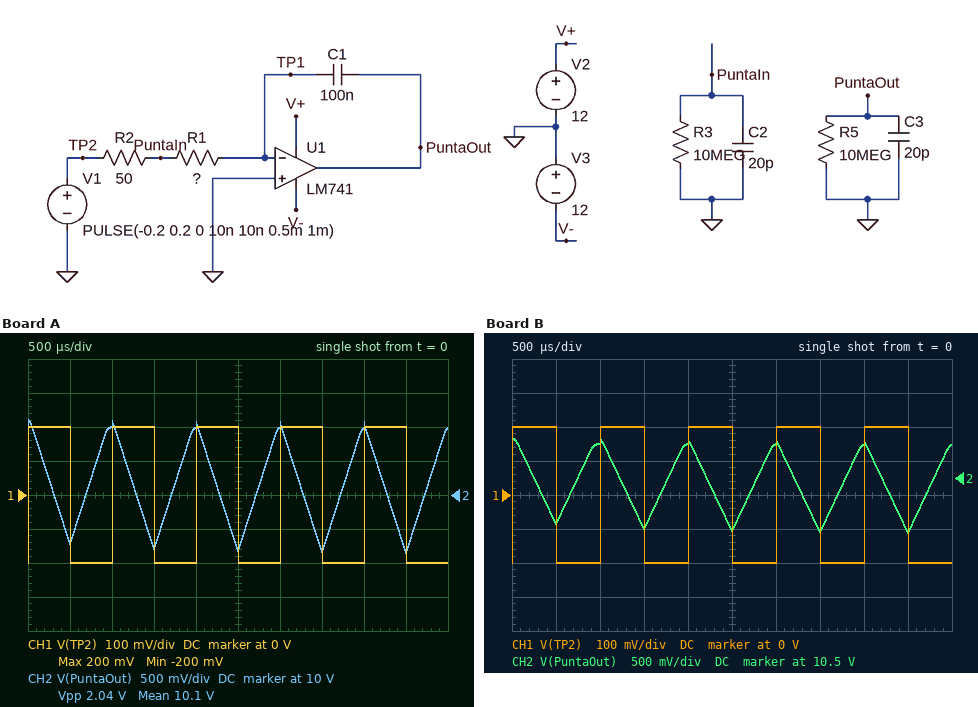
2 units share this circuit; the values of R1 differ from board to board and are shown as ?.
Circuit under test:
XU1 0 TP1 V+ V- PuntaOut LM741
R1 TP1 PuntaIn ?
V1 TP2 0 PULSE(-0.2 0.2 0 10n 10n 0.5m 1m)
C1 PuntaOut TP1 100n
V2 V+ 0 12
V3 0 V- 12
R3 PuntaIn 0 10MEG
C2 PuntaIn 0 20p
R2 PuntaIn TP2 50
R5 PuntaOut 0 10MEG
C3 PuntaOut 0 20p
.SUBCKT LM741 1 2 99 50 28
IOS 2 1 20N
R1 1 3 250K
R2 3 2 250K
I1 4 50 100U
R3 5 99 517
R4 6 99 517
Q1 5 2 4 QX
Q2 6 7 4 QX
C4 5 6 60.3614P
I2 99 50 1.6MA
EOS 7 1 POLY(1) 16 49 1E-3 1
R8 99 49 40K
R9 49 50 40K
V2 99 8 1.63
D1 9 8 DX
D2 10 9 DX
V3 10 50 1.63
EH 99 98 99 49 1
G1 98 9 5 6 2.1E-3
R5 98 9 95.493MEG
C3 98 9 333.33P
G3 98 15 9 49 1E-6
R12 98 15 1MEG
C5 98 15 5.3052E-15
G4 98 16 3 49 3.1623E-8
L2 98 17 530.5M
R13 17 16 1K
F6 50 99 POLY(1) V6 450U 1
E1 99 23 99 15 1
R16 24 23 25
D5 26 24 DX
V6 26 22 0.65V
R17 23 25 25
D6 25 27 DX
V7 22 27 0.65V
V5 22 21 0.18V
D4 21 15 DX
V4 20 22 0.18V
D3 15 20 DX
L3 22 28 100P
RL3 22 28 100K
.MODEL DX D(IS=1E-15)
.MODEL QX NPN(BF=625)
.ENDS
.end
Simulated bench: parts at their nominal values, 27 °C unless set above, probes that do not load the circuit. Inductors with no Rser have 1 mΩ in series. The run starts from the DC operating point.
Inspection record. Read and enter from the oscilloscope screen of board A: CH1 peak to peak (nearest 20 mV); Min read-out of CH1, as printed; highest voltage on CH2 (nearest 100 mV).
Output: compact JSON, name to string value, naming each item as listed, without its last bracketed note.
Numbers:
{"CH1 peak to peak": "400 mV", "Min read-out of CH1, as printed": "-200 mV", "highest voltage on CH2": "11.1 V"}
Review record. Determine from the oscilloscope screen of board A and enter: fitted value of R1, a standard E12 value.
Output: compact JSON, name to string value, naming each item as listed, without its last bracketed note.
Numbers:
{"fitted value of R1, a standard E12 value": "470 Ω"}
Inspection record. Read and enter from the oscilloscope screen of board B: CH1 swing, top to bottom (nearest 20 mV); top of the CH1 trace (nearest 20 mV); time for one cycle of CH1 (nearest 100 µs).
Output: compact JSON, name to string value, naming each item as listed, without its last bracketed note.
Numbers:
{"CH1 swing, top to bottom": "400 mV", "top of the CH1 trace": "200 mV", "time for one cycle of CH1": "1.0 ms"}
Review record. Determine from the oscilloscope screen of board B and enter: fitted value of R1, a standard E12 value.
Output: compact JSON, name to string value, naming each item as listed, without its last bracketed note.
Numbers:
{"fitted value of R1, a standard E12 value": "680 Ω"}
